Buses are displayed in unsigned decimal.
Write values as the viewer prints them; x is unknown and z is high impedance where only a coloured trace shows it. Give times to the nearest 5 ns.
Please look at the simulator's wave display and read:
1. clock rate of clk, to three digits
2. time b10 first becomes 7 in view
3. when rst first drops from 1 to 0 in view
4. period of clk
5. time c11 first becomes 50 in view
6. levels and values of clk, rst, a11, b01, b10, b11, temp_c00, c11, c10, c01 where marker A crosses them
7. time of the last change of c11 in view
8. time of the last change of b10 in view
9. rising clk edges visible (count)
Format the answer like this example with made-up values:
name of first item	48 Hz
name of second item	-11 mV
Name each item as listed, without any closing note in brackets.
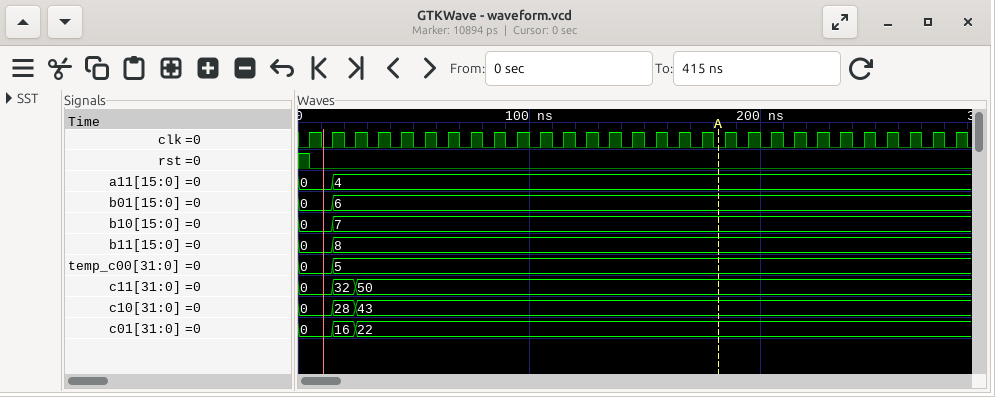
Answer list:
clock rate of clk, to three digits	100 MHz
time b10 first becomes 7 in view	15 ns
when rst first drops from 1 to 0 in view	5 ns
period of clk	10 ns
time c11 first becomes 50 in view	25 ns
levels and values of clk, rst, a11, b01, b10, b11, temp_c00, c11, c10, c01 where marker A crosses them	clk=0, rst=0, a11=4, b01=6, b10=7, b11=8, temp_c00=5, c11=50, c10=43, c01=22
time of the last change of c11 in view	25 ns
time of the last change of b10 in view	15 ns
rising clk edges visible	29
